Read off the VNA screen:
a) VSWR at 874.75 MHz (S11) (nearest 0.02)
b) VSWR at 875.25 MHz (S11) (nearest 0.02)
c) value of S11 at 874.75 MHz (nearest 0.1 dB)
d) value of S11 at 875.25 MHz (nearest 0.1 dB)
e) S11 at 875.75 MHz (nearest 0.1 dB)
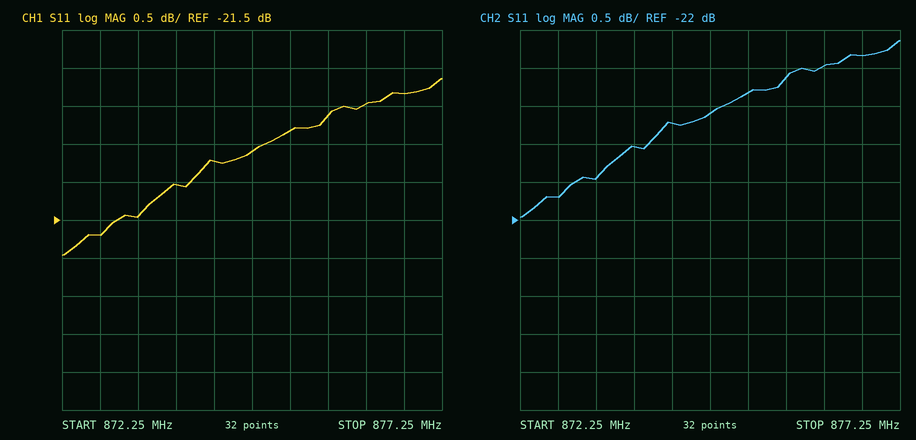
1.20
1.22
-20.6 dB
-20.3 dB
-20.1 dB
